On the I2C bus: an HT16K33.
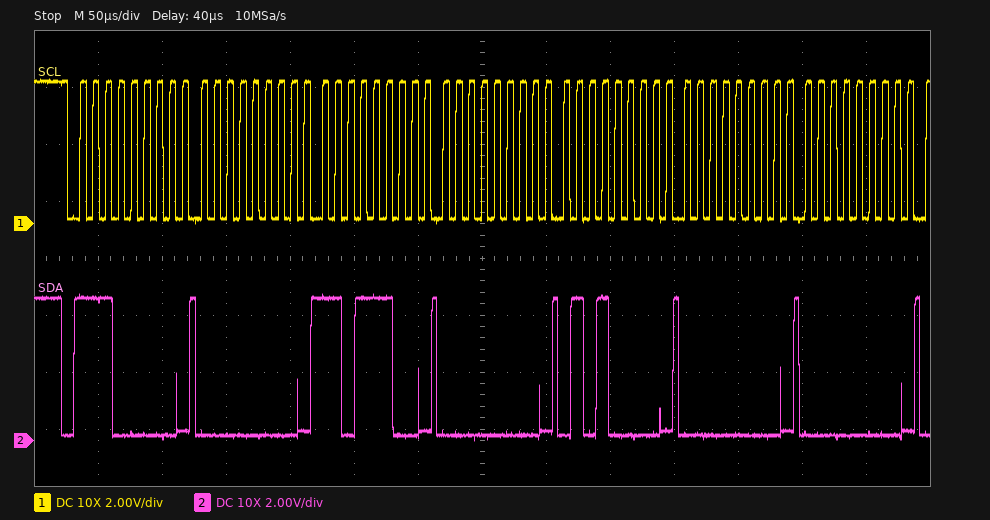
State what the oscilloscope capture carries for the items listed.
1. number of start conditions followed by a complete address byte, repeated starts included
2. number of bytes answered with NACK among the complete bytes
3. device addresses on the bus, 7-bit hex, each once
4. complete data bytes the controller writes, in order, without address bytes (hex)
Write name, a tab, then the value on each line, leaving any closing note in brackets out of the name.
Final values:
number of start conditions followed by a complete address byte, repeated starts included	1
number of bytes answered with NACK among the complete bytes	0
device addresses on the bus, 7-bit hex, each once	0x70
complete data bytes the controller writes, in order, without address bytes	00 DC 00 50 00 00
